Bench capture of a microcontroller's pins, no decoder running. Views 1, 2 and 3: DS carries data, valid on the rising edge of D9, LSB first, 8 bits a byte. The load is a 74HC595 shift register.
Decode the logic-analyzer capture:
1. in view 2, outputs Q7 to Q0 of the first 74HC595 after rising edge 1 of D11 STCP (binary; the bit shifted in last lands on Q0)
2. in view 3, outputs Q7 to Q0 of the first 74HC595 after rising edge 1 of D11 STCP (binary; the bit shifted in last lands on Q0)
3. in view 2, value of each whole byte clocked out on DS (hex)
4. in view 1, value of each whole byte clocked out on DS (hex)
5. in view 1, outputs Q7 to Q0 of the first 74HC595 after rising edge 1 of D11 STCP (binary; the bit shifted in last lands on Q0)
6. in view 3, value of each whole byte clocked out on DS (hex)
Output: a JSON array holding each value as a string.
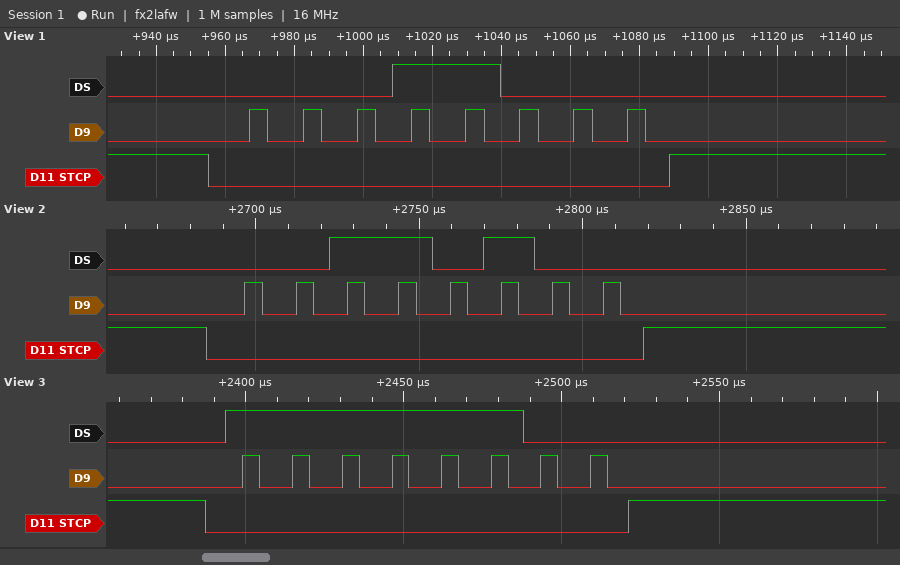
["00110100", "11111100", "2C", "0x18", "00011000", "3F"]
